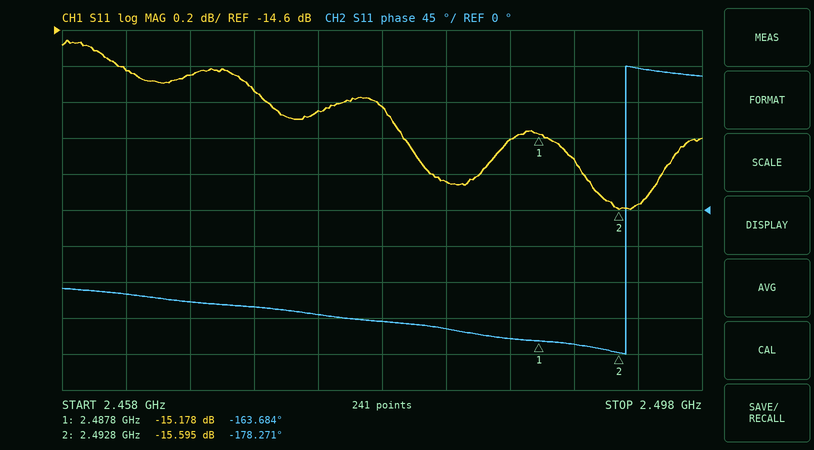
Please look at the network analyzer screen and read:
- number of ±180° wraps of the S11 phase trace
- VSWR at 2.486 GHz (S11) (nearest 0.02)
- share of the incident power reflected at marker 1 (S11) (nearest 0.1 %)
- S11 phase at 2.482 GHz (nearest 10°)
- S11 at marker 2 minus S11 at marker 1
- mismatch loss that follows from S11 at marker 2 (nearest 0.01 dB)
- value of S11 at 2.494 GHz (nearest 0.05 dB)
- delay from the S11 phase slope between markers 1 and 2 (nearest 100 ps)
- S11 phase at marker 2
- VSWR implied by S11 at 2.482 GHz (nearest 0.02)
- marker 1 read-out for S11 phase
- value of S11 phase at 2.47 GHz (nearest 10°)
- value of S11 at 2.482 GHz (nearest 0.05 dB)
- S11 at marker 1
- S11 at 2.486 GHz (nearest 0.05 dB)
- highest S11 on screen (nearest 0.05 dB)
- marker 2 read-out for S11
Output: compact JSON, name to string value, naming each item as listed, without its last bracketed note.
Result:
{"number of ±180° wraps of the S11 phase trace": "1", "VSWR at 2.486 GHz (S11)": "1.42", "share of the incident power reflected at marker 1 (S11)": "3.0 %", "S11 phase at 2.482 GHz": "-150°", "S11 at marker 2 minus S11 at marker 1": "-0.417 dB", "mismatch loss that follows from S11 at marker 2": "0.12 dB", "value of S11 at 2.494 GHz": "-15.55 dB", "delay from the S11 phase slope between markers 1 and 2": "8.1 ns", "S11 phase at marker 2": "-178.271°", "VSWR implied by S11 at 2.482 GHz": "1.40", "marker 1 read-out for S11 phase": "-163.684°", "value of S11 phase at 2.47 GHz": "-120°", "value of S11 at 2.482 GHz": "-15.45 dB", "S11 at marker 1": "-15.178 dB", "S11 at 2.486 GHz": "-15.20 dB", "highest S11 on screen": "-14.65 dB", "marker 2 read-out for S11": "-15.595 dB"}
